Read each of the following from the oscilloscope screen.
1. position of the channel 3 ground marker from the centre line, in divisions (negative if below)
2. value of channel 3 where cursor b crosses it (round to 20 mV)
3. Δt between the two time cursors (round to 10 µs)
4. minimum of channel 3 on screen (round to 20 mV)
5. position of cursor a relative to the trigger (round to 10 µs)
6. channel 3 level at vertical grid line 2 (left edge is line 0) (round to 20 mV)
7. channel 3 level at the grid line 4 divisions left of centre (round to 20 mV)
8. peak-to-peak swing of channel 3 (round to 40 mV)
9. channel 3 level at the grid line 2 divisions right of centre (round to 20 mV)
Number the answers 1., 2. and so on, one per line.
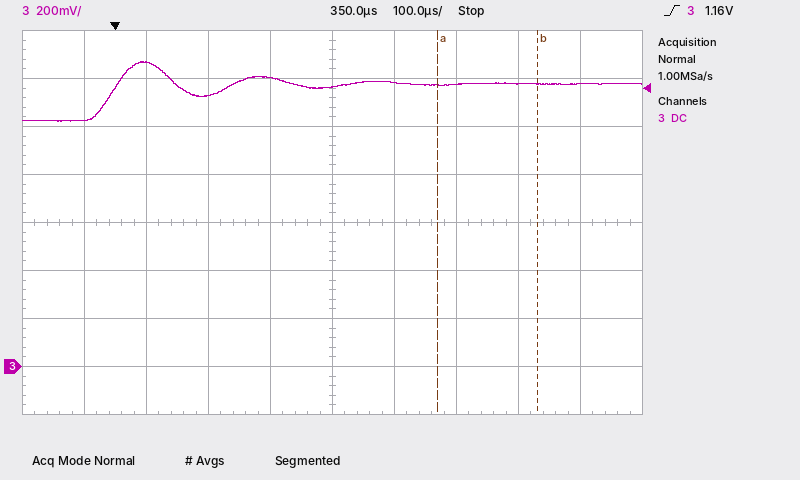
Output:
1. -3.0 div
2. 1.18 V
3. 160 µs
4. 1.02 V
5. +520 µs
6. 1.26 V
7. 1.02 V
8. 240 mV
9. 1.18 V
